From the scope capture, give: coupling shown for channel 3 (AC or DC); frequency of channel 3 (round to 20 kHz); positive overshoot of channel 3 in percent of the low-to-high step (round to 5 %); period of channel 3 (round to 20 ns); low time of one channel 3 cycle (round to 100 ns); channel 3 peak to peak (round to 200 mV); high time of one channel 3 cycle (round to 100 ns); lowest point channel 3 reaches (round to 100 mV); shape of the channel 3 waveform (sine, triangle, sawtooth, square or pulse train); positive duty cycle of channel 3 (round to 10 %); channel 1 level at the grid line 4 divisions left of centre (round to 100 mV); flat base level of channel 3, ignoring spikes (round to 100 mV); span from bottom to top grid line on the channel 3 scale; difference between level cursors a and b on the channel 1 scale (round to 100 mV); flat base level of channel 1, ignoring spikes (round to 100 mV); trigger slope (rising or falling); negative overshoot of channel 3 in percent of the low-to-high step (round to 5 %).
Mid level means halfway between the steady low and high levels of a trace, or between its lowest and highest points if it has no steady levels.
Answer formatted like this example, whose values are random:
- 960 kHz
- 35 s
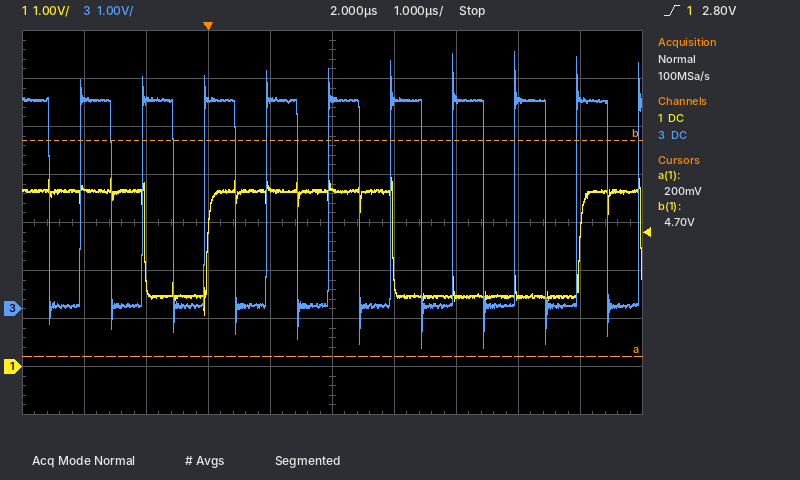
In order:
- DC
- 1.00 MHz
- 25 %
- 1.00 µs
- 500 ns
- 6.2 V
- 500 ns
- -800 mV
- square
- 50 %
- 3.7 V
- 100 mV
- 8 V
- 4.5 V
- 1.5 V
- rising
- 20 %
